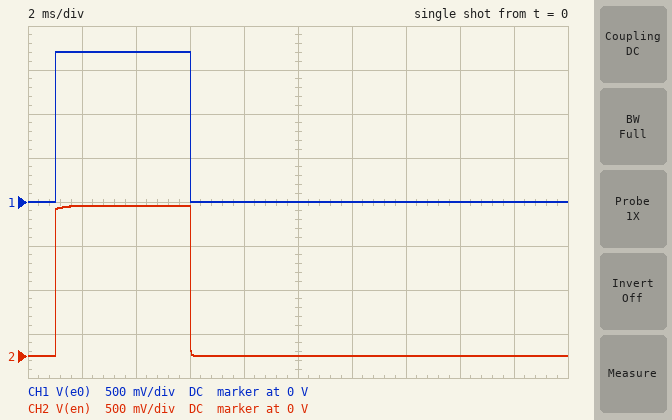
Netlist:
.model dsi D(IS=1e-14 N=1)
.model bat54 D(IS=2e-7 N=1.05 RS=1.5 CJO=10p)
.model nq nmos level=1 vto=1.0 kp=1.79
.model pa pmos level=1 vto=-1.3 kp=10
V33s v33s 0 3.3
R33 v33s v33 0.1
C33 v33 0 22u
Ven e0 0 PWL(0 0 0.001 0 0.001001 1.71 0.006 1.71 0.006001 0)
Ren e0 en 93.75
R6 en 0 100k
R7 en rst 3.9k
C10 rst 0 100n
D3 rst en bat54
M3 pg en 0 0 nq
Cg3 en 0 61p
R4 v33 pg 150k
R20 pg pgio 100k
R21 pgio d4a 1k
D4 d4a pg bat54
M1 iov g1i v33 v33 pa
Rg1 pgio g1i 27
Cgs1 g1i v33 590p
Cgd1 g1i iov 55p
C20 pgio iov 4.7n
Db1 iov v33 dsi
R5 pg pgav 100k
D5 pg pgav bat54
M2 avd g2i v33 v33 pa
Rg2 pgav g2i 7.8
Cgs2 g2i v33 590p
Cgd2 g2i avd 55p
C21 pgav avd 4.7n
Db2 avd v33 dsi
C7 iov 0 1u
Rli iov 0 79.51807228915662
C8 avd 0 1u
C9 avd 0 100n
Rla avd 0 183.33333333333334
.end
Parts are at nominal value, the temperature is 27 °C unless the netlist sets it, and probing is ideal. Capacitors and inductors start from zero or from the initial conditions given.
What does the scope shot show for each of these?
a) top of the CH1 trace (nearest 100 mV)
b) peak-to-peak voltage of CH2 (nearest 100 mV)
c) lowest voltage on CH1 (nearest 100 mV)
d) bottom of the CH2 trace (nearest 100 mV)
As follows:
1.7 V
1.7 V
0 V
0 V
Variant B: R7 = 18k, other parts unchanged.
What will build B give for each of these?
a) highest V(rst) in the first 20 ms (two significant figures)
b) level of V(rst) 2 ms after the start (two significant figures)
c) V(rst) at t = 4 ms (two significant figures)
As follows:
1.6 V
730 mV
1.4 V
